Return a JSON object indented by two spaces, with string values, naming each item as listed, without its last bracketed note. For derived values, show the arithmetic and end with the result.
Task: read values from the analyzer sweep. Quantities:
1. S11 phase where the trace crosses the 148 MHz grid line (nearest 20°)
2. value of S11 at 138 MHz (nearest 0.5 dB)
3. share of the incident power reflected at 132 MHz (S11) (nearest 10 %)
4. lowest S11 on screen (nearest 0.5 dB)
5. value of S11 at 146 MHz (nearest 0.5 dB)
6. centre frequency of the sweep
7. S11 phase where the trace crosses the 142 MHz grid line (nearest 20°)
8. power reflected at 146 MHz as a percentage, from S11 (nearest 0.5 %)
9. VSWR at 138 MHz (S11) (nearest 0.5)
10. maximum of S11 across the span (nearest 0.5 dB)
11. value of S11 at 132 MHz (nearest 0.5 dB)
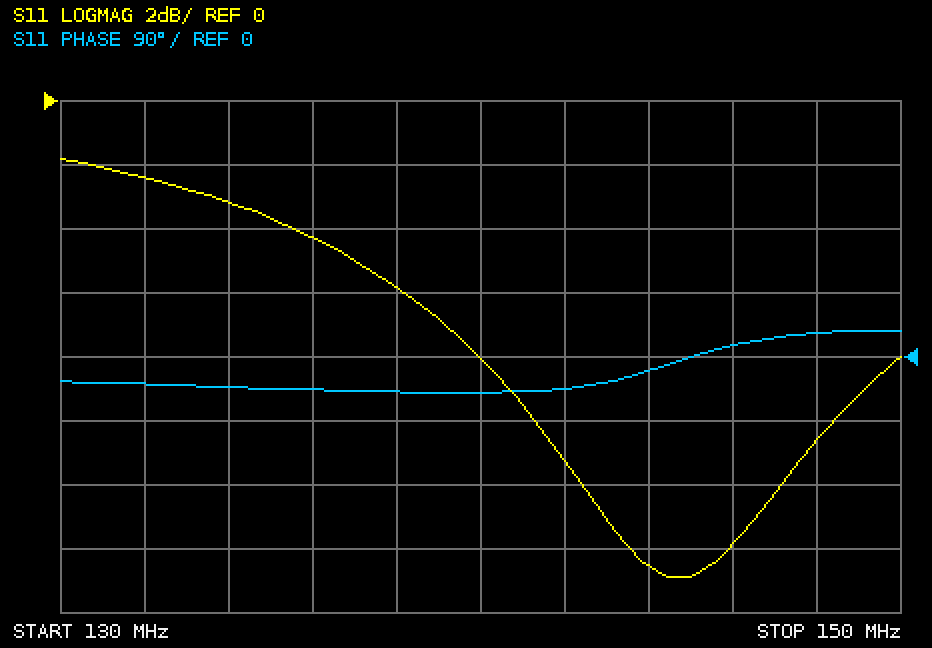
{
  "S11 phase where the trace crosses the 148 MHz grid line": "40°",
  "value of S11 at 138 MHz": "-6.0 dB",
  "share of the incident power reflected at 132 MHz (S11)": "10^(-2.5/10) ≈ 56.2 %, so 60 % to the nearest 10 %",
  "lowest S11 on screen": "-15.0 dB",
  "value of S11 at 146 MHz": "-14.0 dB",
  "centre frequency of the sweep": "140 MHz",
  "S11 phase where the trace crosses the 142 MHz grid line": "-40°",
  "power reflected at 146 MHz as a percentage, from S11": "10^(-14/10) ≈ 4.0 %",
  "VSWR at 138 MHz (S11)": "|Γ| = 10^(-6/20) = 0.5012; VSWR = (1 + 0.5012)/(1 − 0.5012) ≈ 3.0",
  "maximum of S11 across the span": "-2.0 dB",
  "value of S11 at 132 MHz": "-2.5 dB"
}
